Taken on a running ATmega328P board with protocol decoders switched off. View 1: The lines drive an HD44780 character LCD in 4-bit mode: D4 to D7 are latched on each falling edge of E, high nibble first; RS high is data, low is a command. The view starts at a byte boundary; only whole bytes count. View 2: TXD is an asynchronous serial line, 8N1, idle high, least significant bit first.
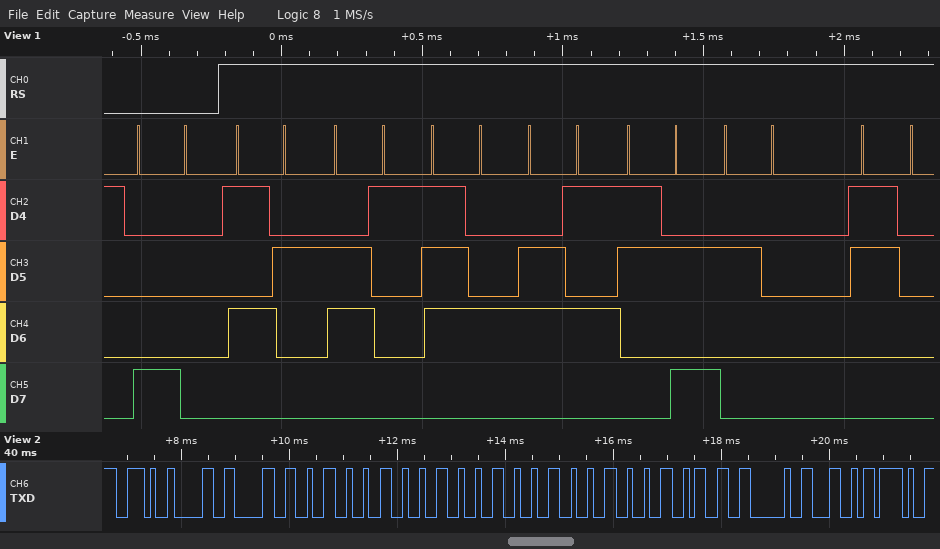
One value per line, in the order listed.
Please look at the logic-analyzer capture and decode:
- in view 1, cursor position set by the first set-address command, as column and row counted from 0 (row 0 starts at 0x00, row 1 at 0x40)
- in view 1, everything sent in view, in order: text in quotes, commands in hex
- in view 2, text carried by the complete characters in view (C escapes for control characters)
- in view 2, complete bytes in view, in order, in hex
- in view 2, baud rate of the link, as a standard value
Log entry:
column 0, row 0
0x80 "Rate: 0"
".0022222223 L/"
2E 30 30 32 32 32 32 32 32 32 33 20 4C 2F
9600 baud
